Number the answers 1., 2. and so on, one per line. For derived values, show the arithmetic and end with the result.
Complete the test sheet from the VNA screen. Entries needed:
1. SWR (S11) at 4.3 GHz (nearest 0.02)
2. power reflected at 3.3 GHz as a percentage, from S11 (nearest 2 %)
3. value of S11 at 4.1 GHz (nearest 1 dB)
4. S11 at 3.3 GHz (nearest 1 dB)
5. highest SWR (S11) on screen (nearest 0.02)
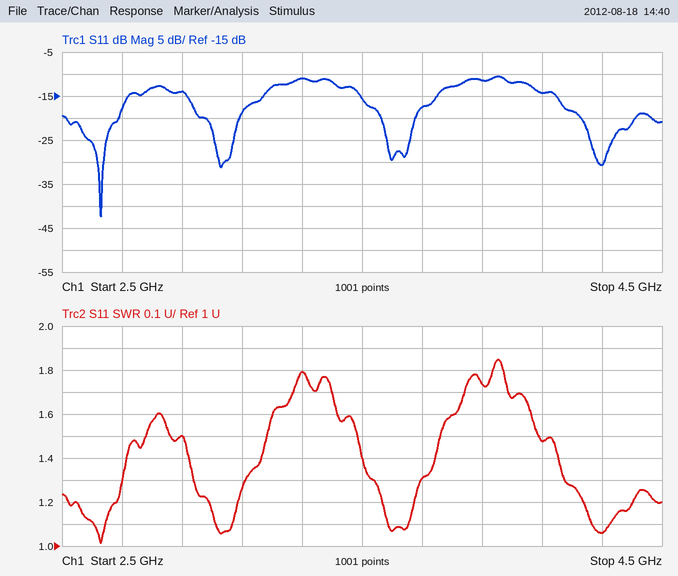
1. 1.06
2. 10^(-11/10) ≈ 8 %
3. -14 dB
4. -11 dB
5. 1.84
